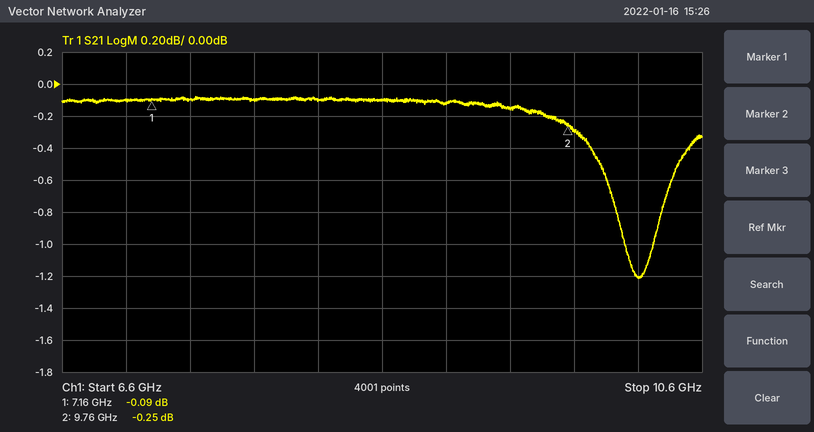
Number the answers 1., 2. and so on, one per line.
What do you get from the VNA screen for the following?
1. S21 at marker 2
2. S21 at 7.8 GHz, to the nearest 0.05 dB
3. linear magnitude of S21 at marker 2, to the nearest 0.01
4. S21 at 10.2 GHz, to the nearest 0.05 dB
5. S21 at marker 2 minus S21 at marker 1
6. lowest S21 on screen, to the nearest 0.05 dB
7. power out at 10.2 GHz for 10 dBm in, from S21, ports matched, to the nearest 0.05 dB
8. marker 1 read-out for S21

1. -0.25 dB
2. -0.10 dB
3. 0.97
4. -1.20 dB
5. -0.16 dB
6. -1.20 dB
7. 8.80 dBm
8. -0.09 dB
